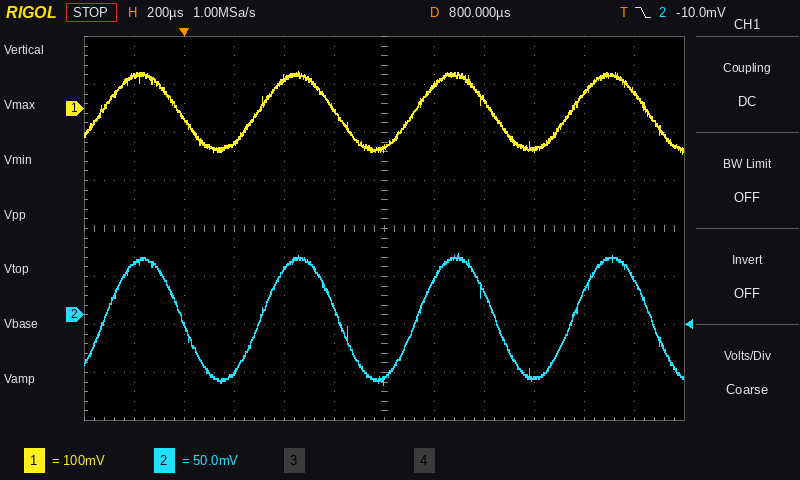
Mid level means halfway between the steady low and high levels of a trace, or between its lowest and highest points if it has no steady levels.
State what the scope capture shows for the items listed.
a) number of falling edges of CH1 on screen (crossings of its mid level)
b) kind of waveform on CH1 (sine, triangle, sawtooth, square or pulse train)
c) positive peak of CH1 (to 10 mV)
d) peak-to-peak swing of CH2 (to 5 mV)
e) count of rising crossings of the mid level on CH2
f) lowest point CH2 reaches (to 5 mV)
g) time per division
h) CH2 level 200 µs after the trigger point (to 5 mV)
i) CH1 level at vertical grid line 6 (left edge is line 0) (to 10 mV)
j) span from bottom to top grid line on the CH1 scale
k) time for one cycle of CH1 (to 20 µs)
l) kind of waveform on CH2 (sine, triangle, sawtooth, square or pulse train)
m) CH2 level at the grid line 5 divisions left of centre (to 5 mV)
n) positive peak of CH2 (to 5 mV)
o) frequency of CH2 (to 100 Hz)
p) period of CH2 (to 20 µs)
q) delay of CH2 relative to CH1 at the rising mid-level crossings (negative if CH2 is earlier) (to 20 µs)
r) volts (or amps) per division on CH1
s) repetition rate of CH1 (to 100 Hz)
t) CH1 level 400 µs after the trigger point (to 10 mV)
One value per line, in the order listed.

4
sine
80 mV
135 mV
4
-70 mV
200 µs
-60 mV
-80 mV
800 mV
620 µs
sine
55 mV
65 mV
1.6 kHz
620 µs
+20 µs
100 mV
1.6 kHz
60 mV
